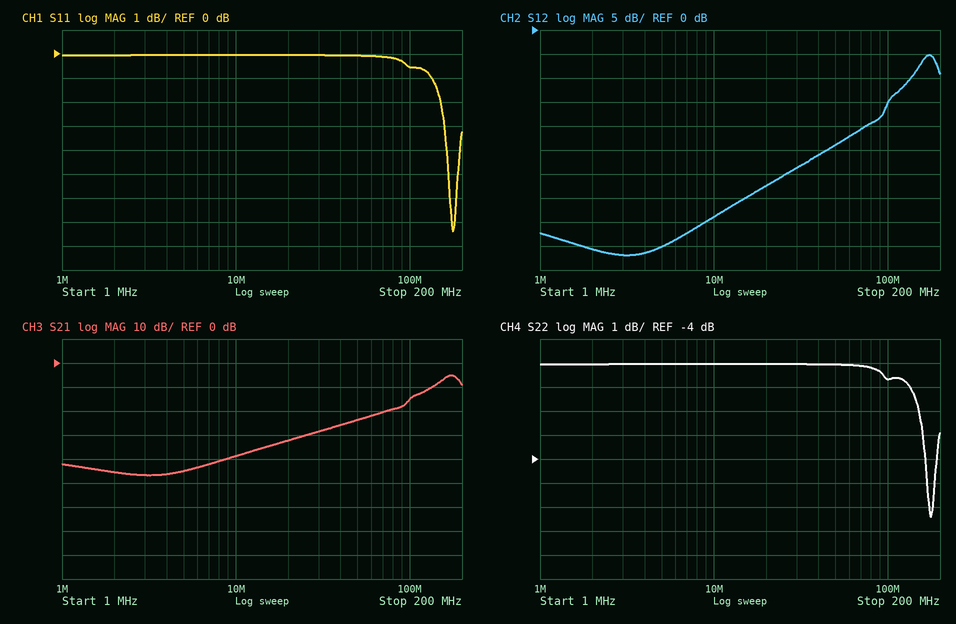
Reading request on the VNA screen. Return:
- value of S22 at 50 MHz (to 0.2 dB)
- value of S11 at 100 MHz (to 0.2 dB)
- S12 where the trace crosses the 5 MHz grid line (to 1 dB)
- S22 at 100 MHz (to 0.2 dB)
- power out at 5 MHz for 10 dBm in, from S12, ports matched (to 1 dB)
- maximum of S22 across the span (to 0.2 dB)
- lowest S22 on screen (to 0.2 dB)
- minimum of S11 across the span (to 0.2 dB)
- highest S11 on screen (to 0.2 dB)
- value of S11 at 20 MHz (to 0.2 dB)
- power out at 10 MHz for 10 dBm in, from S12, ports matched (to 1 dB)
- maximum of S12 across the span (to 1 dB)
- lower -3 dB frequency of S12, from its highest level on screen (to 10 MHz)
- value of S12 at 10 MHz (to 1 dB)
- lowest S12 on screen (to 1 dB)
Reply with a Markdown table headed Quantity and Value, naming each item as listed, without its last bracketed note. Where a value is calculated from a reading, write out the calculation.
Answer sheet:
| Quantity | Value |
|---|---|
| value of S22 at 50 MHz | 0.0 dB |
| value of S11 at 100 MHz | -0.6 dB |
| S12 where the trace crosses the 5 MHz grid line | -45 dB |
| S22 at 100 MHz | -0.6 dB |
| power out at 5 MHz for 10 dBm in, from S12, ports matched | 10 dBm + (-45 dB) = -35 dBm |
| maximum of S22 across the span | 0.0 dB |
| lowest S22 on screen | -6.4 dB |
| minimum of S11 across the span | -7.4 dB |
| highest S11 on screen | 0.0 dB |
| value of S11 at 20 MHz | 0.0 dB |
| power out at 10 MHz for 10 dBm in, from S12, ports matched | 10 dBm + (-39 dB) = -29 dBm |
| maximum of S12 across the span | -5 dB |
| lower -3 dB frequency of S12, from its highest level on screen | 150 MHz |
| value of S12 at 10 MHz | -39 dB |
| lowest S12 on screen | -47 dB |
